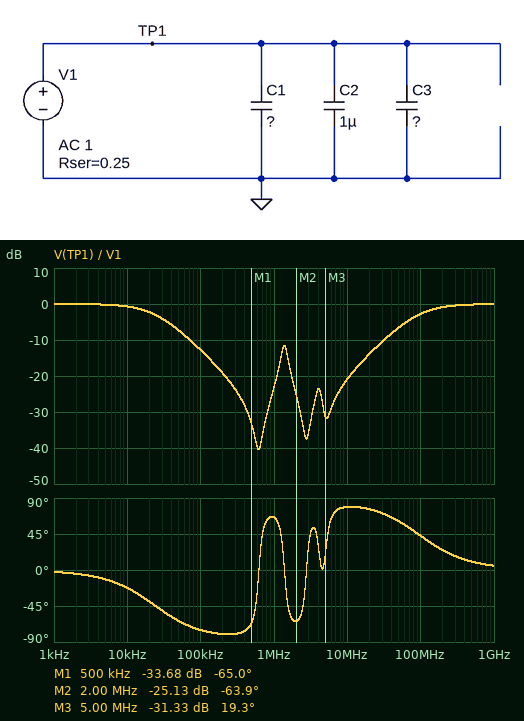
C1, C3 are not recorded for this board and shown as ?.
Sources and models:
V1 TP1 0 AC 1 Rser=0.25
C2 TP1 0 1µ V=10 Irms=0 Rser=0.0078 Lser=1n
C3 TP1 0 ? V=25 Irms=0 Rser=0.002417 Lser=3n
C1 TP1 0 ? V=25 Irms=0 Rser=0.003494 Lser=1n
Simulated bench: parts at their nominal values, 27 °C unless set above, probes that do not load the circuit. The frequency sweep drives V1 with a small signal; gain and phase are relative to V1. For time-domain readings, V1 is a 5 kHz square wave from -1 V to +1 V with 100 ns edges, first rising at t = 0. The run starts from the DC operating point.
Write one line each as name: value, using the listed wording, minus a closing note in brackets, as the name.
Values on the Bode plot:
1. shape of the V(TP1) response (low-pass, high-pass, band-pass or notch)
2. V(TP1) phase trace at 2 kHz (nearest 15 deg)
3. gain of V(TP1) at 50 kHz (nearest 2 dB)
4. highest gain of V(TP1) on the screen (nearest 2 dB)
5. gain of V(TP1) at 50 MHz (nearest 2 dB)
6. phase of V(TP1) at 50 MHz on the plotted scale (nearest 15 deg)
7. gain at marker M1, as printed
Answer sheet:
shape of the V(TP1) response: notch
V(TP1) phase trace at 2 kHz: 0 deg
gain of V(TP1) at 50 kHz: -8 dB
highest gain of V(TP1) on the screen: 0 dB
gain of V(TP1) at 50 MHz: -6 dB
phase of V(TP1) at 50 MHz on the plotted scale: 60 deg
gain at marker M1, as printed: -33.68 dB
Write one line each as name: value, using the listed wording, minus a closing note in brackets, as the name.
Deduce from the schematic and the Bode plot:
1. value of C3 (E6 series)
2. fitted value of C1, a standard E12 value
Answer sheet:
value of C3: 22 µF
fitted value of C1, a standard E12 value: 3.3 µF
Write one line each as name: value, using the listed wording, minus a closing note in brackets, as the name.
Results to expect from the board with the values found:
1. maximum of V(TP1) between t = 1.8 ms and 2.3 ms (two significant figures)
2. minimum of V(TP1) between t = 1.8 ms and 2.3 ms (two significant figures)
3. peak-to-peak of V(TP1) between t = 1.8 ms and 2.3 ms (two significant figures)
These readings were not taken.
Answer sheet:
maximum of V(TP1) between t = 1.8 ms and 2.3 ms: 1.0 V
minimum of V(TP1) between t = 1.8 ms and 2.3 ms: -1.0 V
peak-to-peak of V(TP1) between t = 1.8 ms and 2.3 ms: 2.0 V
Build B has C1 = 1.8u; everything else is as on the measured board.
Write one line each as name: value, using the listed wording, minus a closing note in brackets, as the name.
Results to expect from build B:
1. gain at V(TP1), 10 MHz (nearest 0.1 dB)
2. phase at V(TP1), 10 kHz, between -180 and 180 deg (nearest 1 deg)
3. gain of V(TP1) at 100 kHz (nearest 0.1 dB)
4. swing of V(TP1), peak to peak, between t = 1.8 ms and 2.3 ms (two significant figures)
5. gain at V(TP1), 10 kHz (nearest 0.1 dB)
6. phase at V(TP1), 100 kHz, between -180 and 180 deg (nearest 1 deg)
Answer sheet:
gain at V(TP1), 10 MHz: -21.1 dB
phase at V(TP1), 10 kHz, between -180 and 180 deg: -21 deg
gain of V(TP1) at 100 kHz: -12.3 dB
swing of V(TP1), peak to peak, between t = 1.8 ms and 2.3 ms: 2.0 V
gain at V(TP1), 10 kHz: -0.6 dB
phase at V(TP1), 100 kHz, between -180 and 180 deg: -74 deg
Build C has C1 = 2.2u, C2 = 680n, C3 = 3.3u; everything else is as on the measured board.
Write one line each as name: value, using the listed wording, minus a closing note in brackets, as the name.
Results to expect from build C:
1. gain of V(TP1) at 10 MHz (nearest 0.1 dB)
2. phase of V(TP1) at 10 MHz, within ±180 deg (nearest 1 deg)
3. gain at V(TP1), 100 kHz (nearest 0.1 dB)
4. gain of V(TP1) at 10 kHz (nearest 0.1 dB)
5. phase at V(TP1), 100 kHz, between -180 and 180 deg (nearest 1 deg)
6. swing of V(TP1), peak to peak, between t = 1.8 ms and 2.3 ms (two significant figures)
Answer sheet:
gain of V(TP1) at 10 MHz: -21.7 dB
phase of V(TP1) at 10 MHz, within ±180 deg: 78 deg
gain at V(TP1), 100 kHz: -2.9 dB
gain of V(TP1) at 10 kHz: 0 dB
phase at V(TP1), 100 kHz, between -180 and 180 deg: -44 deg
swing of V(TP1), peak to peak, between t = 1.8 ms and 2.3 ms: 2.0 V
